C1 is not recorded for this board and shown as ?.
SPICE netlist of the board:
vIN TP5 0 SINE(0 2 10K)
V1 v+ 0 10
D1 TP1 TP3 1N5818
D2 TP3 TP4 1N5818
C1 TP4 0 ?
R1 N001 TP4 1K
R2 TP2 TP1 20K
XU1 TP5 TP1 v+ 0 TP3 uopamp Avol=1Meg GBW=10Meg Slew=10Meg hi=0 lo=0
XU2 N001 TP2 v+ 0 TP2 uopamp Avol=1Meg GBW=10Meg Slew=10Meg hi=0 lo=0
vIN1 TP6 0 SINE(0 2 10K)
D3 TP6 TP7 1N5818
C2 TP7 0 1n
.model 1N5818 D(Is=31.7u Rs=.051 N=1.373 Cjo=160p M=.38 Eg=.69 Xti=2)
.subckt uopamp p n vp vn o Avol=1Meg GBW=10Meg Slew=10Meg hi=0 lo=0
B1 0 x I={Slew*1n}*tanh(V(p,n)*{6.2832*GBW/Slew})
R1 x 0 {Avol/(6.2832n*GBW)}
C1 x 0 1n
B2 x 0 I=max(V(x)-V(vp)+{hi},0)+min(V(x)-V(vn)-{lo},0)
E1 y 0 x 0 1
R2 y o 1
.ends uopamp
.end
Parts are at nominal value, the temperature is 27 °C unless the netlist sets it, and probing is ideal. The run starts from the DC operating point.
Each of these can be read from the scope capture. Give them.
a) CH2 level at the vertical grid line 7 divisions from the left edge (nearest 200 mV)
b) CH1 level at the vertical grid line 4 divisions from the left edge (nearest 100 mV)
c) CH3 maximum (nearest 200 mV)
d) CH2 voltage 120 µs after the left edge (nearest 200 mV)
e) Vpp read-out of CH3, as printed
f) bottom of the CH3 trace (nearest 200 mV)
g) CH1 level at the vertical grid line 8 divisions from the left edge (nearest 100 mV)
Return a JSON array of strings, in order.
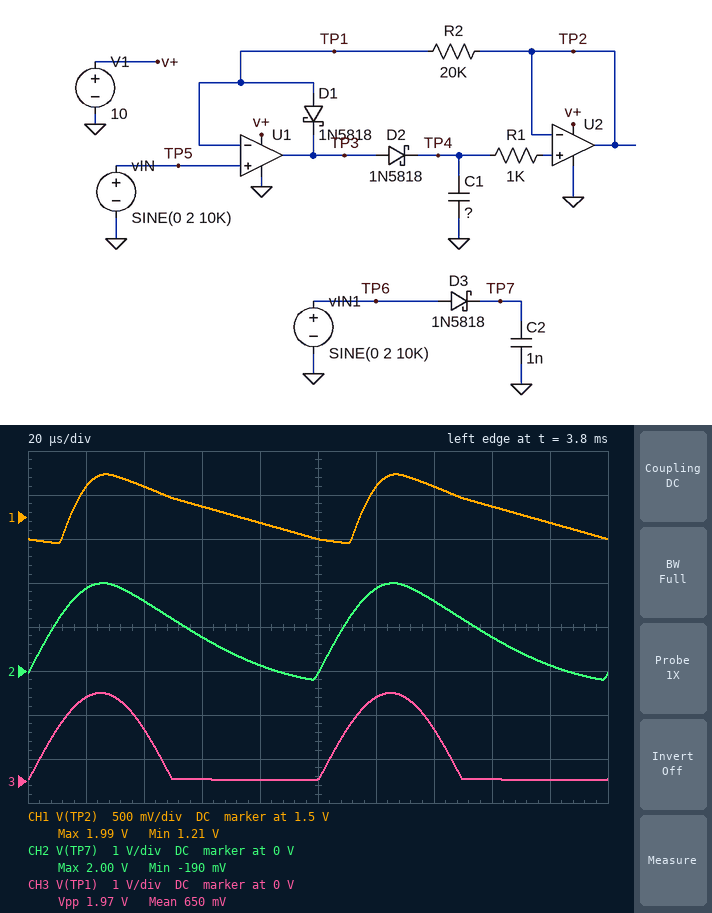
["1.6 V", "1.4 V", "2.0 V", "1.8 V", "1.97 V", "0 V", "1.6 V"]
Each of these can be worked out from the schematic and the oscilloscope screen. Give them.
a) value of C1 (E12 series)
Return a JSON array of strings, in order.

["3.3 nF"]
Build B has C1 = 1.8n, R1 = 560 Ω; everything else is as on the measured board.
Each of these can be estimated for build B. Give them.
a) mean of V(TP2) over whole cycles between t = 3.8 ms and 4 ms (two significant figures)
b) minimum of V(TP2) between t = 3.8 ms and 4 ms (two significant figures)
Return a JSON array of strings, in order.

["1.3 V", "650 mV"]
